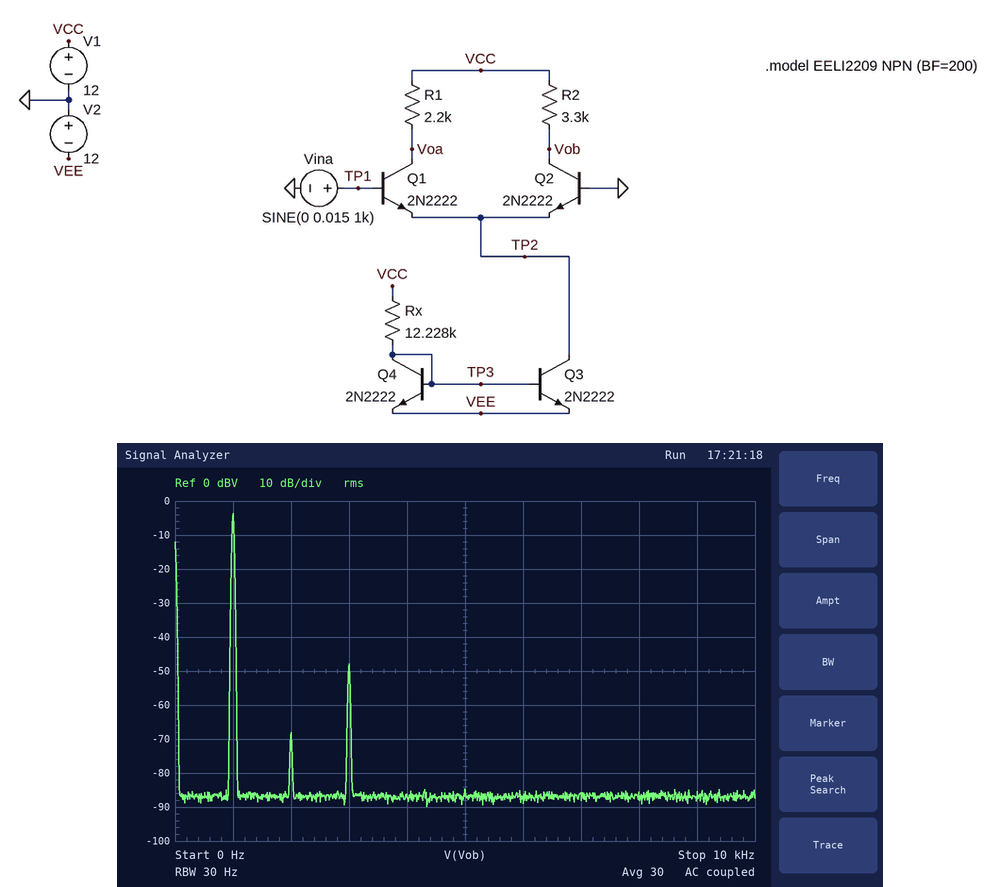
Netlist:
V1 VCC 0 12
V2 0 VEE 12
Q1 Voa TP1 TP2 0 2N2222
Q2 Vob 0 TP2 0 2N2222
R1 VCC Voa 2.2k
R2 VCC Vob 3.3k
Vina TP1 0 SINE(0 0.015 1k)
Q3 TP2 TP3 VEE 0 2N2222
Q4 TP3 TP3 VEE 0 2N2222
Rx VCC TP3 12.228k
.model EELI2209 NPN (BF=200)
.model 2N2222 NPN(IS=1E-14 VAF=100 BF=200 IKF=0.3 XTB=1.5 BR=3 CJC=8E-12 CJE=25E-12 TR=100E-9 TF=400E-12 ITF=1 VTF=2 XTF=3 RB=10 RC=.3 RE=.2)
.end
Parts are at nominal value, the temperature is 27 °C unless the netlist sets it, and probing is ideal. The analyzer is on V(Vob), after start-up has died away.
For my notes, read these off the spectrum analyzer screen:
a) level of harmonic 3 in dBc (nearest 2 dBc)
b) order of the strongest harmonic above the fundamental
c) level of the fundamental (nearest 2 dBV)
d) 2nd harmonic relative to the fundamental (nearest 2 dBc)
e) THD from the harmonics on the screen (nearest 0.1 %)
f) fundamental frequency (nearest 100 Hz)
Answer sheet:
-44 dBc
3
-4 dBV
-64 dBc
0.6 %
1.0 kHz
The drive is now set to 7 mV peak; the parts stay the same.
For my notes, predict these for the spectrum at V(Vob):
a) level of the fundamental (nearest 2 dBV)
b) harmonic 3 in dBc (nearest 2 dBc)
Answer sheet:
-10 dBV
-58 dBc
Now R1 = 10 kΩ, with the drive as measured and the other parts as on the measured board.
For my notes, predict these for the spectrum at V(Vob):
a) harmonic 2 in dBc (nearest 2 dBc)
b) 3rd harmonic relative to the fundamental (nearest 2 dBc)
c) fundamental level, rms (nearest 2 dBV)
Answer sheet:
-44 dBc
-38 dBc
-4 dBV
